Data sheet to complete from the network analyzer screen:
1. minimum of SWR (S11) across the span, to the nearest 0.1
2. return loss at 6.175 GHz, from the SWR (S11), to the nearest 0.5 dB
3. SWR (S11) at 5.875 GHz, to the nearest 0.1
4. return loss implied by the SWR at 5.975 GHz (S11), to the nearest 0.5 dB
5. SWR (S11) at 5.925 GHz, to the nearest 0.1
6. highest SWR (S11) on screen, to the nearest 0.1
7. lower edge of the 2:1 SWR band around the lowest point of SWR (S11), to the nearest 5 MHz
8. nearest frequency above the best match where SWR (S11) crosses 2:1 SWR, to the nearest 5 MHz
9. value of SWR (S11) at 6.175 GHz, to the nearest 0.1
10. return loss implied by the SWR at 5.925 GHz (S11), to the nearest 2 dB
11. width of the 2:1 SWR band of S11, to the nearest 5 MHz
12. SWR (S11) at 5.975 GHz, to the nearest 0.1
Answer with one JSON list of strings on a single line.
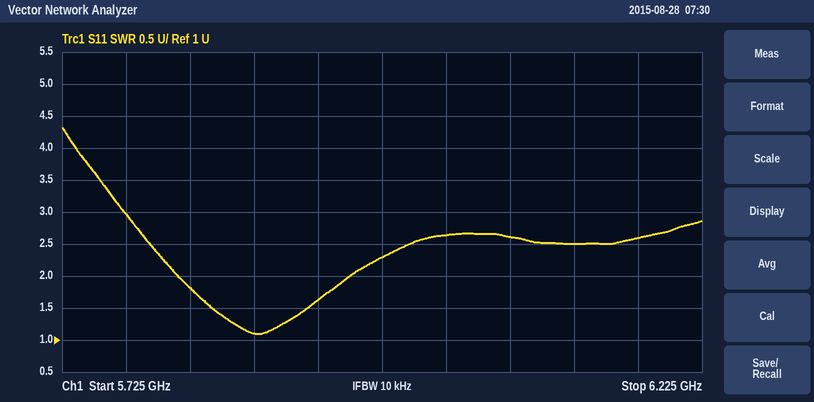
["1.1", "7.0 dB", "1.1", "8.0 dB", "1.6", "4.3", "5.815 GHz", "5.950 GHz", "2.6", "12 dB", "135 MHz", "2.3"]
